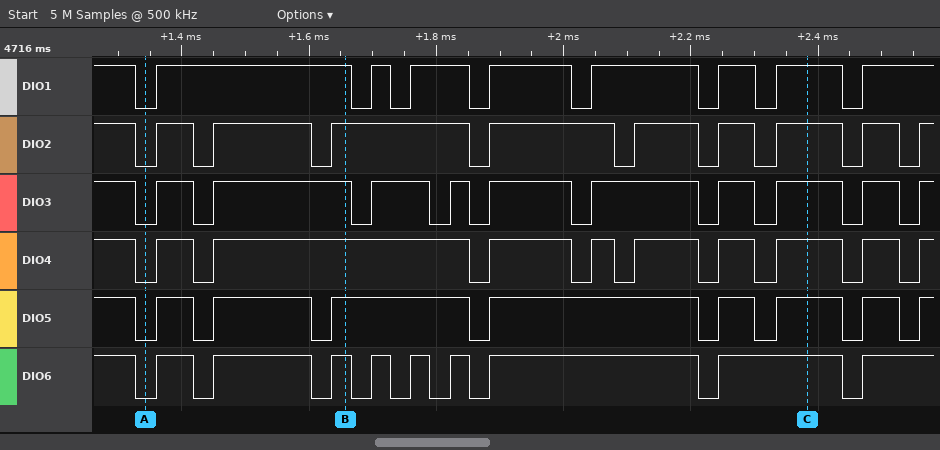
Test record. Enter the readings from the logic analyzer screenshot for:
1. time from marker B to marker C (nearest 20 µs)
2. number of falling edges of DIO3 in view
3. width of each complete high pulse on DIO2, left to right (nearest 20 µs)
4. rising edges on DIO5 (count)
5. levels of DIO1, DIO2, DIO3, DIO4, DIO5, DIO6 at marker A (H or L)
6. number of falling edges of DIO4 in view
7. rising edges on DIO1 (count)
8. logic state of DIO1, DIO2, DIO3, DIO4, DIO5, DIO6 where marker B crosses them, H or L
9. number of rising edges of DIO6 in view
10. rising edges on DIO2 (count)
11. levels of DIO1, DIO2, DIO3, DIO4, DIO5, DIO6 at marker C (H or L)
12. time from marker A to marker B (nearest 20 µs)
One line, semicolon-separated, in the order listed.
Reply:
720 µs; 10; 60 µs, 160 µs, 220 µs, 200 µs, 100 µs, 60 µs, 100 µs, 60 µs; 8; DIO1=L, DIO2=L, DIO3=L, DIO4=L, DIO5=L, DIO6=L; 9; 8; DIO1=H, DIO2=H, DIO3=H, DIO4=H, DIO5=H, DIO6=H; 9; 9; DIO1=H, DIO2=H, DIO3=H, DIO4=H, DIO5=H, DIO6=H; 320 µs
